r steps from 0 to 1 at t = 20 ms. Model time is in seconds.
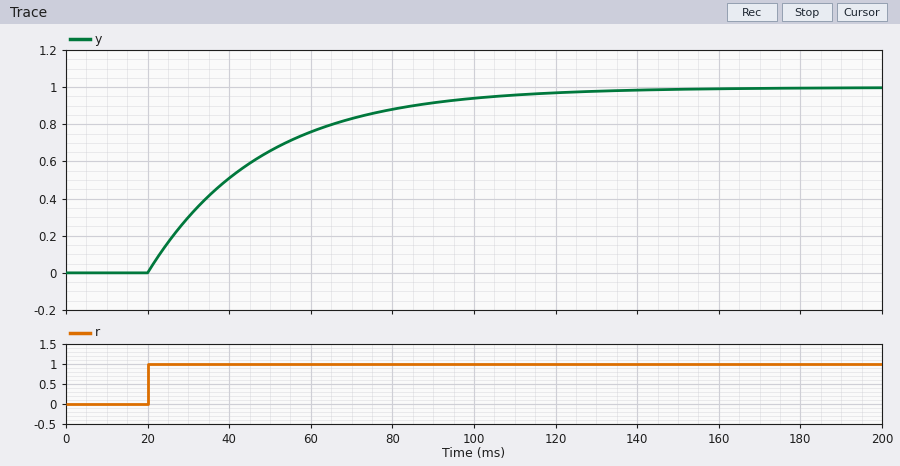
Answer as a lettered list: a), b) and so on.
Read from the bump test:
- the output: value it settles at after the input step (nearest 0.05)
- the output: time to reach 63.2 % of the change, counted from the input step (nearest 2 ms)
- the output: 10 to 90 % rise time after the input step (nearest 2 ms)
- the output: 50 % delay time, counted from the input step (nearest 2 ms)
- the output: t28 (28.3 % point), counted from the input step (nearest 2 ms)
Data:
a) 1.00
b) 28 ms
c) 62 ms
d) 20 ms
e) 10 ms
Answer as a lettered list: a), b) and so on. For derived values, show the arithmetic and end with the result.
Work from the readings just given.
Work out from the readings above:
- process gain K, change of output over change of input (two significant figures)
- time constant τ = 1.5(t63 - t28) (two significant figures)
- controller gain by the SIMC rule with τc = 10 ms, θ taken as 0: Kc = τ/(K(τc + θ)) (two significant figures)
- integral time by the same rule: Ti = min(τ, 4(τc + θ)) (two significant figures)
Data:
a) (1 - 0) / 1 = 1.0
b) 1.5 × (28 - 10) = 27 ms
c) 27 / (1 × (10 + 0)) = 2.7
d) min(27, 4 × (10 + 0)) = 27 ms
